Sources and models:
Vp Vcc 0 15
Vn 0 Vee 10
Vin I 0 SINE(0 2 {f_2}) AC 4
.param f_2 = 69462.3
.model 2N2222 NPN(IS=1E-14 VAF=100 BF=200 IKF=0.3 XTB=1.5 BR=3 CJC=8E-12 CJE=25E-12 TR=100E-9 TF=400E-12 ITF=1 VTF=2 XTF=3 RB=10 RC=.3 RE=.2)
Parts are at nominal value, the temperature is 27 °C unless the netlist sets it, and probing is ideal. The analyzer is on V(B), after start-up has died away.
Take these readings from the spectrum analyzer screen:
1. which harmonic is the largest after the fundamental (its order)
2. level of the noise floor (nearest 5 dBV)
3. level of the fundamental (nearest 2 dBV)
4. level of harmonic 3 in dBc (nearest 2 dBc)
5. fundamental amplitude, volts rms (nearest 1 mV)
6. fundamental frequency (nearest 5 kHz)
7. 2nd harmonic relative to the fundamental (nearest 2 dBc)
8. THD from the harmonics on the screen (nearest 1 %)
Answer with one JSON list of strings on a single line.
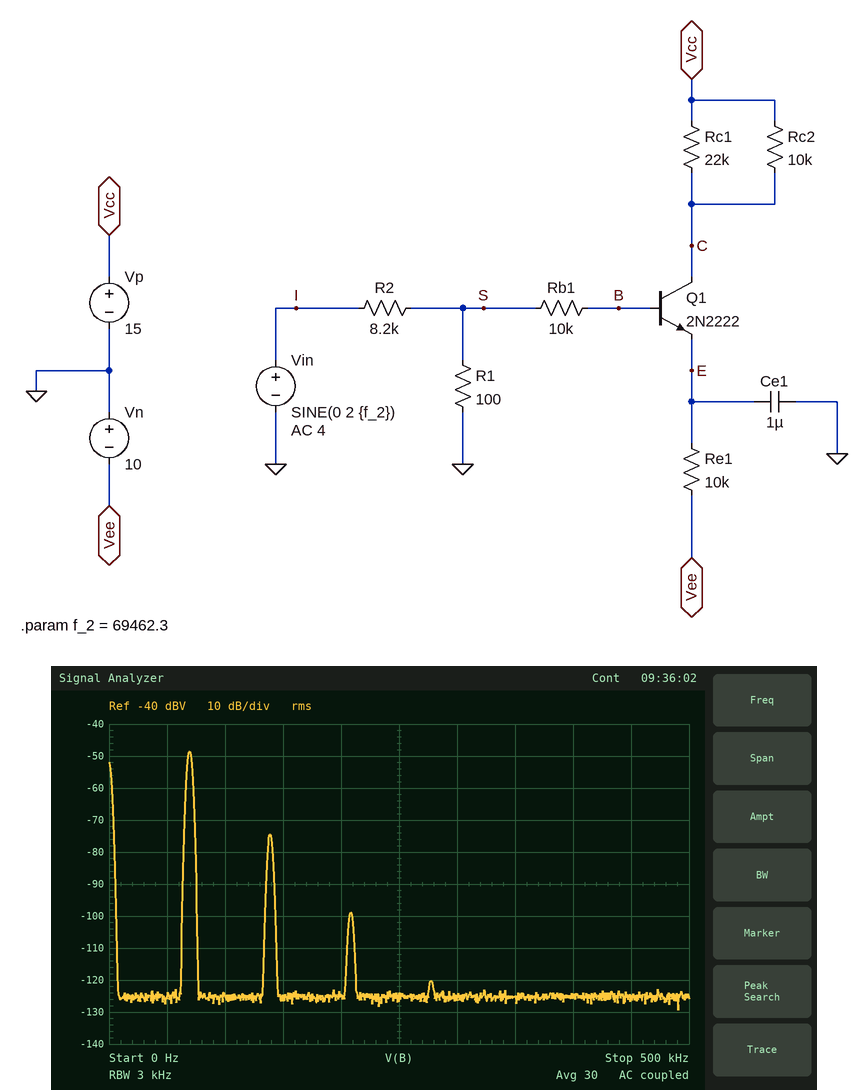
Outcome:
["2", "-125 dBV", "-48 dBV", "-50 dBc", "4 mV", "70 kHz", "-26 dBc", "5 %"]
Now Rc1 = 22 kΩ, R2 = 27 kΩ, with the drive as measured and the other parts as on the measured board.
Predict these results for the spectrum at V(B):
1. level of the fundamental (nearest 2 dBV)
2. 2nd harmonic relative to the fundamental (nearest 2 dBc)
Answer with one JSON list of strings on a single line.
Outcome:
["-58 dBV", "-36 dBc"]
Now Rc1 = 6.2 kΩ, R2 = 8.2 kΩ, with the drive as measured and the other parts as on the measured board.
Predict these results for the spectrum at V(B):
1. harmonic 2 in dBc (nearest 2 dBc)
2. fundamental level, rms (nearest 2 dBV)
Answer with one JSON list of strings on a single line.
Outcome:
["-24 dBc", "-46 dBV"]
